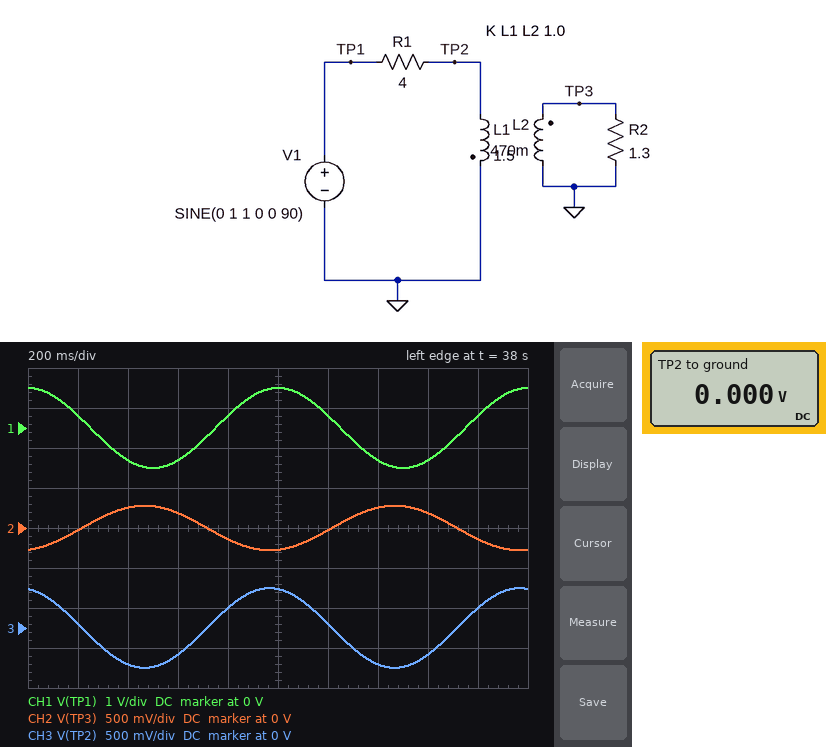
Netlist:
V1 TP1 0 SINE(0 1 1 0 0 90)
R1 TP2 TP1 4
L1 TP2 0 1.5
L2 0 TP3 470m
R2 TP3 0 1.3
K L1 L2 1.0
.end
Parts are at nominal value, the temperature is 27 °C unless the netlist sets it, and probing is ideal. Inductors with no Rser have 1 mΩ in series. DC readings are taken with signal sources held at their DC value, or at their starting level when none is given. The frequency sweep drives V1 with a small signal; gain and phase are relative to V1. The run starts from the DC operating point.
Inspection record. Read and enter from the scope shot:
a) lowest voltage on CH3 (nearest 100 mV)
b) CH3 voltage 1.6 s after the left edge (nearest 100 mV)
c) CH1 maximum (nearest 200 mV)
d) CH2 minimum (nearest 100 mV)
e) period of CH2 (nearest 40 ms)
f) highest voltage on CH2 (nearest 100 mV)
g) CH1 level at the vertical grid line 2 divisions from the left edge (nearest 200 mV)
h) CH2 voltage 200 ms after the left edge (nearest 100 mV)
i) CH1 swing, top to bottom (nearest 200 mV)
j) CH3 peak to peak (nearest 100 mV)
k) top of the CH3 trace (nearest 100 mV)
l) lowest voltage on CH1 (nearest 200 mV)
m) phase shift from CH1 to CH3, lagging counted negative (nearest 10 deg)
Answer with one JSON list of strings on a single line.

["-500 mV", "-300 mV", "1.0 V", "-300 mV", "1.00 s", "300 mV", "-800 mV", "0 V", "2.0 V", "1.0 V", "500 mV", "-1.0 V", "10 deg"]
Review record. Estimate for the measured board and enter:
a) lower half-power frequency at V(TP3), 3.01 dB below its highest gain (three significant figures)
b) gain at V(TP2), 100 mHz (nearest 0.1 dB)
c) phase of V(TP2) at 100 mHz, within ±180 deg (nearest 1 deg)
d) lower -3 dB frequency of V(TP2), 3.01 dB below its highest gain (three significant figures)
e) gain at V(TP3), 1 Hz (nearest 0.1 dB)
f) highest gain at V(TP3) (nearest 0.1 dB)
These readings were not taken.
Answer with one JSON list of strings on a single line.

["216 mHz", "-13.4 dB", "65 deg", "216 mHz", "-11.1 dB", "-10.9 dB"]
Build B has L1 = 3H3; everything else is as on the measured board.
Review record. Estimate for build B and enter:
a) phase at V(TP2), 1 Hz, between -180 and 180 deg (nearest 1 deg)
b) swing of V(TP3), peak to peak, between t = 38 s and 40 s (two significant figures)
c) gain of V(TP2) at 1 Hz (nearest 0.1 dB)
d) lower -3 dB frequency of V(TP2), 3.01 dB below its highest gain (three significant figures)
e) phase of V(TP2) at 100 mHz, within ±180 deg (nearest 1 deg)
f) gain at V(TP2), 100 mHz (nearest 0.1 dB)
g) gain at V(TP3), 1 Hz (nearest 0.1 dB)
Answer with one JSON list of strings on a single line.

["8 deg", "520 mV", "-3.2 dB", "134 mHz", "53 deg", "-7.6 dB", "-11.7 dB"]
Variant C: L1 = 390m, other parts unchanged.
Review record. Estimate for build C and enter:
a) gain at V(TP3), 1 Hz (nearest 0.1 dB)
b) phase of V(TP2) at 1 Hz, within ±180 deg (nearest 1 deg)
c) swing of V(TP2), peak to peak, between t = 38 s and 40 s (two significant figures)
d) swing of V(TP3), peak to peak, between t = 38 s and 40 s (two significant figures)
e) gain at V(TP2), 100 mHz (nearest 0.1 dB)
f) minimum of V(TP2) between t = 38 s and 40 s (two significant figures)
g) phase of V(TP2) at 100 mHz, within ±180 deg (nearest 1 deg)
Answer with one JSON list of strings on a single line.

["-13.1 dB", "19 deg", "400 mV", "440 mV", "-24.6 dB", "-200 mV", "74 deg"]
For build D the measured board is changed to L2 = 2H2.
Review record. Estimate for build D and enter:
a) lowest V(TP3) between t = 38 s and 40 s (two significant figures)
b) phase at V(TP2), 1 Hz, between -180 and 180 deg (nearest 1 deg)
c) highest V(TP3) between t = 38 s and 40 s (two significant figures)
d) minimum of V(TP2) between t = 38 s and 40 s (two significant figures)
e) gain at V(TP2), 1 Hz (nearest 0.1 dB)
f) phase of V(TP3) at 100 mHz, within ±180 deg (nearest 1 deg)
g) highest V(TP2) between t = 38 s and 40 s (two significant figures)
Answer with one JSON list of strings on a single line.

["-220 mV", "4 deg", "220 mV", "-180 mV", "-14.8 dB", "-142 deg", "180 mV"]
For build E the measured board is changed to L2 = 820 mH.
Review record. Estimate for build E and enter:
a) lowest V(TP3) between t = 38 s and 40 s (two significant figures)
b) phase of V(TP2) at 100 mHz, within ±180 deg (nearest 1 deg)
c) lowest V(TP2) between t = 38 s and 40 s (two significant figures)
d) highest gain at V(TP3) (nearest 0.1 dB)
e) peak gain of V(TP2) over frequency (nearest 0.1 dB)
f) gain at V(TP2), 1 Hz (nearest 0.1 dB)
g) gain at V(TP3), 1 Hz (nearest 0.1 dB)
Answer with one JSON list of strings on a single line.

["-270 mV", "58 deg", "-370 mV", "-11.2 dB", "-8.6 dB", "-8.7 dB", "-11.3 dB"]
